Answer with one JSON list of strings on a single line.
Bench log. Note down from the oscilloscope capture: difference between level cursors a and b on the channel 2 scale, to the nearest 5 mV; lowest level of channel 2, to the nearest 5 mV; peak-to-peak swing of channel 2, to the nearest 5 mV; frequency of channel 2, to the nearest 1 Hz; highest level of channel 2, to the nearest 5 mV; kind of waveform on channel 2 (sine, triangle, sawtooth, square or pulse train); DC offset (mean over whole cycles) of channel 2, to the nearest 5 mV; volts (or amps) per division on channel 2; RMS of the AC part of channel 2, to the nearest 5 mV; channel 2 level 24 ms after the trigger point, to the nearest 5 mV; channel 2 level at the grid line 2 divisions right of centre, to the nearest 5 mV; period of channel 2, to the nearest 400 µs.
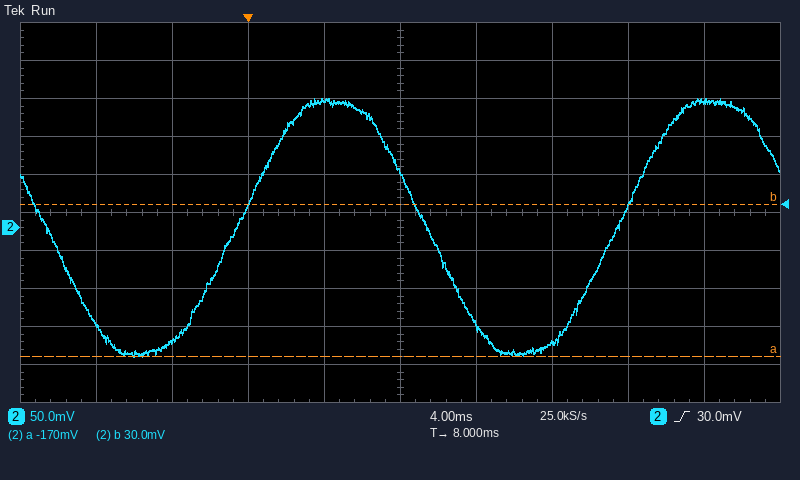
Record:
["200 mV", "-170 mV", "340 mV", "50 Hz", "170 mV", "sine", "0 mV", "50 mV", "120 mV", "165 mV", "-150 mV", "20.0 ms"]
